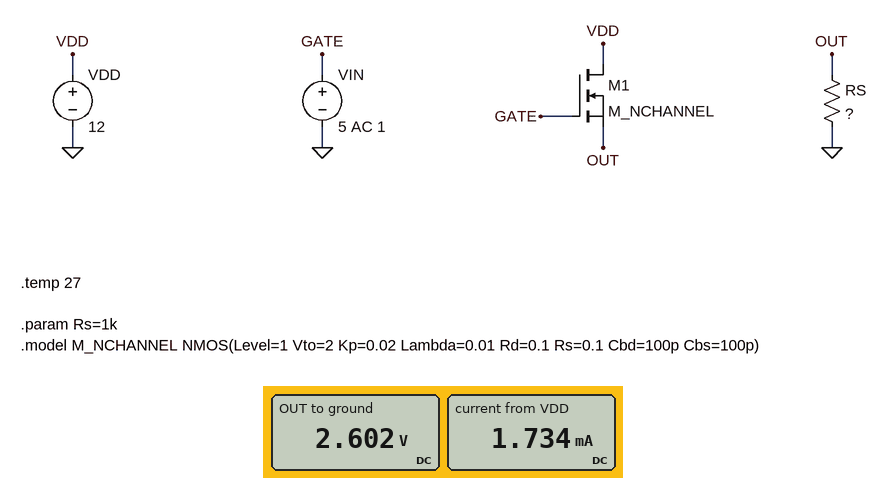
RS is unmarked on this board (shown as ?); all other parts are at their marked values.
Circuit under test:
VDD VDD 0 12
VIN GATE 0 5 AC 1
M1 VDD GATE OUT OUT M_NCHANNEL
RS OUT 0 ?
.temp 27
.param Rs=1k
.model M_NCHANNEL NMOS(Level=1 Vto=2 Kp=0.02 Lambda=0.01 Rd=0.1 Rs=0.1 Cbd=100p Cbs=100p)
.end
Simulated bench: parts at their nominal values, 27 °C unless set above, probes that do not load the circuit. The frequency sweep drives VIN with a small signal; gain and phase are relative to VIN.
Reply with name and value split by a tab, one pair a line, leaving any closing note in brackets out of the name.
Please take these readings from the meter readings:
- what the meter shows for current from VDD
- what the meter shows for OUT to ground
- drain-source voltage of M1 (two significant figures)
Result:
what the meter shows for current from VDD	1.734 mA
what the meter shows for OUT to ground	2.602 V
drain-source voltage of M1	9.4 V
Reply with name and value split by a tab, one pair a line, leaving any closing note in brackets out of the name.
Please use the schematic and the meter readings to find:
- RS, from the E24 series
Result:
RS, from the E24 series	1.5 kΩ
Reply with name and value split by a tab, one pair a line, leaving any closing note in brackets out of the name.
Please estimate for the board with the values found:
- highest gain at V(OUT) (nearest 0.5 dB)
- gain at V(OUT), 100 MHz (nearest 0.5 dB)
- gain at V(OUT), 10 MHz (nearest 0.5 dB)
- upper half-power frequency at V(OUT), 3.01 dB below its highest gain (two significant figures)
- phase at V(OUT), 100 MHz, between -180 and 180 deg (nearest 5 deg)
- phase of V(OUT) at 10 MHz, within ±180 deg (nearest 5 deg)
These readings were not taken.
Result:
highest gain at V(OUT)	-0.5 dB
gain at V(OUT), 100 MHz	-7.0 dB
gain at V(OUT), 10 MHz	-1.0 dB
upper half-power frequency at V(OUT), 3.01 dB below its highest gain	53 MHz
phase at V(OUT), 100 MHz, between -180 and 180 deg	-60 deg
phase of V(OUT) at 10 MHz, within ±180 deg	-10 deg
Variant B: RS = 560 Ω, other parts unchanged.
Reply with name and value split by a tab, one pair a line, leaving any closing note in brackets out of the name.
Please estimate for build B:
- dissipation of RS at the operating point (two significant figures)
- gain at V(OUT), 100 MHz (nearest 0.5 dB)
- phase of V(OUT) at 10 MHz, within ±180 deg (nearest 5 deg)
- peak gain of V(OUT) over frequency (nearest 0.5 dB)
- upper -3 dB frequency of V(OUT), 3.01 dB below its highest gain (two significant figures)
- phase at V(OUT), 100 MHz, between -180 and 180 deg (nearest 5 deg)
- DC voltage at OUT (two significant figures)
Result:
dissipation of RS at the operating point	10 mW
gain at V(OUT), 100 MHz	-4.5 dB
phase of V(OUT) at 10 MHz, within ±180 deg	-5 deg
peak gain of V(OUT) over frequency	-1.0 dB
upper -3 dB frequency of V(OUT), 3.01 dB below its highest gain	89 MHz
phase at V(OUT), 100 MHz, between -180 and 180 deg	-50 deg
DC voltage at OUT	2.4 V
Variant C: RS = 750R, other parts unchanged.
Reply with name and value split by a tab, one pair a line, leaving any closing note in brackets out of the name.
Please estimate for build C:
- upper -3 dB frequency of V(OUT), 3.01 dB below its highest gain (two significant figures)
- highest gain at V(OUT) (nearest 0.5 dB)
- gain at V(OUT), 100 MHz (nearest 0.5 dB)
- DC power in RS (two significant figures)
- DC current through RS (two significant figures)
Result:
upper -3 dB frequency of V(OUT), 3.01 dB below its highest gain	76 MHz
highest gain at V(OUT)	-1.0 dB
gain at V(OUT), 100 MHz	-5.5 dB
DC power in RS	8.0 mW
DC current through RS	3.3 mA
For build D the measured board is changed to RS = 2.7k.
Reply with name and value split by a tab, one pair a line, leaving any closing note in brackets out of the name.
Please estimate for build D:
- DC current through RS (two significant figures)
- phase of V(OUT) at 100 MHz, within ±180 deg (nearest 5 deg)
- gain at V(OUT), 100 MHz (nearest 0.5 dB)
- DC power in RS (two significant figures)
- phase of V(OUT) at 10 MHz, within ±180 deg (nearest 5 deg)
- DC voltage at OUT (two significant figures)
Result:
DC current through RS	1.0 mA
phase of V(OUT) at 100 MHz, within ±180 deg	-70 deg
gain at V(OUT), 100 MHz	-9.0 dB
DC power in RS	2.7 mW
phase of V(OUT) at 10 MHz, within ±180 deg	-15 deg
DC voltage at OUT	2.7 V
